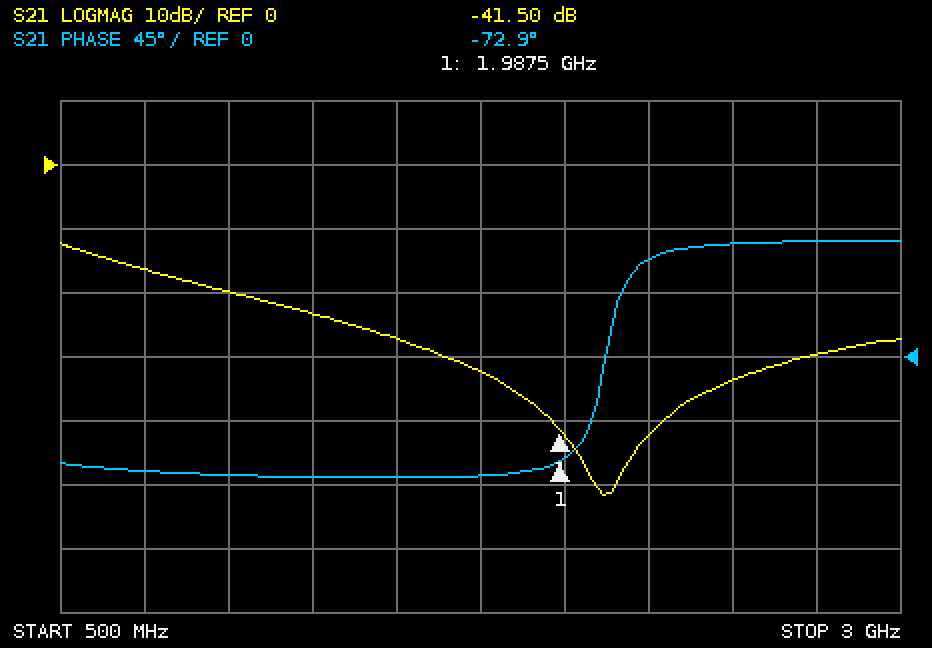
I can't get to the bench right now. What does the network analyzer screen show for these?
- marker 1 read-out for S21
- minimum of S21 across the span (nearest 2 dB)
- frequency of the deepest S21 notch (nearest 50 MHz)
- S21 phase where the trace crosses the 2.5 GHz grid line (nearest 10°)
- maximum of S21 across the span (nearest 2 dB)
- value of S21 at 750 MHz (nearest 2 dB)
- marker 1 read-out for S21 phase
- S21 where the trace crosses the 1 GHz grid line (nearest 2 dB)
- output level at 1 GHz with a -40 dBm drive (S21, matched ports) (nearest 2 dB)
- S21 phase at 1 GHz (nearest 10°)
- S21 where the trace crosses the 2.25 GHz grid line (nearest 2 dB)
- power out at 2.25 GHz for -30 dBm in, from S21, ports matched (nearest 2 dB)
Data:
-41.50 dB
-52 dB
2.10 GHz
80°
-12 dB
-16 dB
-72.9°
-20 dB
-60 dBm
-80°
-42 dB
-72 dBm
